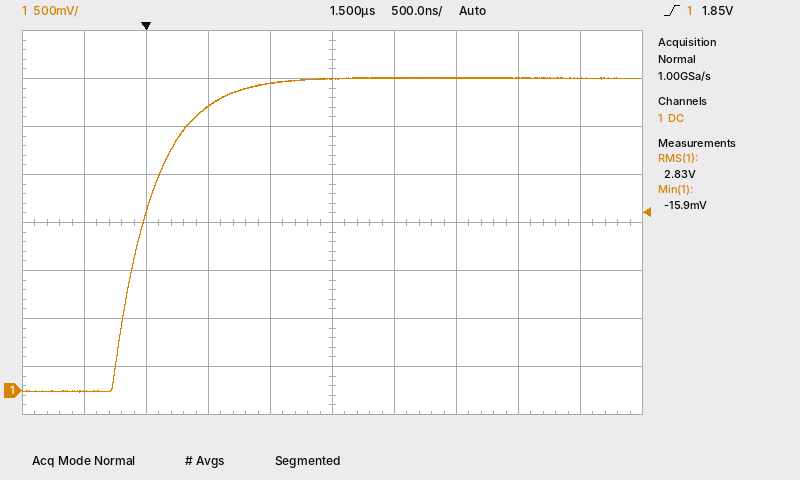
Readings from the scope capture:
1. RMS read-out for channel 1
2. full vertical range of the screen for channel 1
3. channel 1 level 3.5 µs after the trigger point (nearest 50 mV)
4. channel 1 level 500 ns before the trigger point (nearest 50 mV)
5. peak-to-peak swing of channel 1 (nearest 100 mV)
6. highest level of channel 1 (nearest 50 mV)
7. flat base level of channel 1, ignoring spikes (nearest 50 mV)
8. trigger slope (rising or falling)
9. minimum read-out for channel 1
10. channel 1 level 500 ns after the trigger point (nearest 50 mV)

2.83 V
4 V
3.25 V
0 mV
3.30 V
3.25 V
0 mV
rising
-15.9 mV
2.95 V
